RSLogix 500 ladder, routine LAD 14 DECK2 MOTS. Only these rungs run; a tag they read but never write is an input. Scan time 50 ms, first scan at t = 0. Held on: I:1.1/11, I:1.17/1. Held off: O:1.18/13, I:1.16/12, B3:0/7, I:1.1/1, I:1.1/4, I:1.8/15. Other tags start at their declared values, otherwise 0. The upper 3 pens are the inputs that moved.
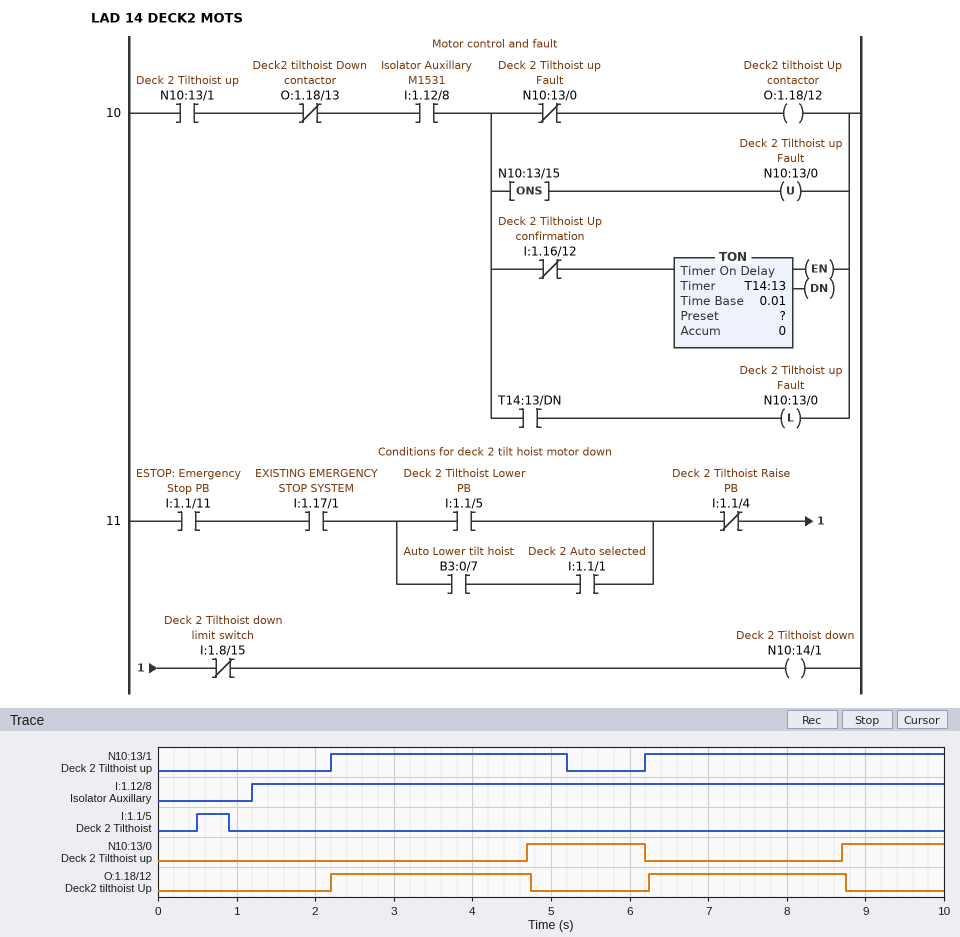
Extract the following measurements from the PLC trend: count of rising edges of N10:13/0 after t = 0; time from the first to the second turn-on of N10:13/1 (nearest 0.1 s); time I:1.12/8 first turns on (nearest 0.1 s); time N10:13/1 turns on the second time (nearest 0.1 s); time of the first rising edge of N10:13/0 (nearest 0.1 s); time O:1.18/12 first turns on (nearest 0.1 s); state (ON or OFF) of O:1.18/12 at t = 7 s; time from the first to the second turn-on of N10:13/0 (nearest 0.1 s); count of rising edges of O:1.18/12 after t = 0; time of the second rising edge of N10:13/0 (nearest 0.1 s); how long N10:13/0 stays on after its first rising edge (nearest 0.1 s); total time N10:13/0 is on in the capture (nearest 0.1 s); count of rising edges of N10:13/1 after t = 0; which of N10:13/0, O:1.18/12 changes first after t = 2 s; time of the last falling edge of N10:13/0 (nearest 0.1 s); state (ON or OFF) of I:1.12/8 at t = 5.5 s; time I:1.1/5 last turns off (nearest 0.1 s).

2
4.0 s
1.2 s
6.2 s
4.7 s
2.2 s
ON
4.0 s
2
8.7 s
1.5 s
2.8 s
2
O:1.18/12
6.2 s
ON
0.9 s
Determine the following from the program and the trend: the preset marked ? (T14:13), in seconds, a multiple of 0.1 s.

2.5 s
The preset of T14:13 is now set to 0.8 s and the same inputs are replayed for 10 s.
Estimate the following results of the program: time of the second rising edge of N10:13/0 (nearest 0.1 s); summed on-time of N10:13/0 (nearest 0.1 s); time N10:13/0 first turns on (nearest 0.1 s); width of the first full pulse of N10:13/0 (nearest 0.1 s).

7.0 s
6.2 s
3.0 s
3.2 s
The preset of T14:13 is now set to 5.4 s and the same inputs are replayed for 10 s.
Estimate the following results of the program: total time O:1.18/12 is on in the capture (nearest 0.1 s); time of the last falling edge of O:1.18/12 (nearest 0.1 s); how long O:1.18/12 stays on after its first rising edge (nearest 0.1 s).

6.8 s
5.2 s
3.0 s
